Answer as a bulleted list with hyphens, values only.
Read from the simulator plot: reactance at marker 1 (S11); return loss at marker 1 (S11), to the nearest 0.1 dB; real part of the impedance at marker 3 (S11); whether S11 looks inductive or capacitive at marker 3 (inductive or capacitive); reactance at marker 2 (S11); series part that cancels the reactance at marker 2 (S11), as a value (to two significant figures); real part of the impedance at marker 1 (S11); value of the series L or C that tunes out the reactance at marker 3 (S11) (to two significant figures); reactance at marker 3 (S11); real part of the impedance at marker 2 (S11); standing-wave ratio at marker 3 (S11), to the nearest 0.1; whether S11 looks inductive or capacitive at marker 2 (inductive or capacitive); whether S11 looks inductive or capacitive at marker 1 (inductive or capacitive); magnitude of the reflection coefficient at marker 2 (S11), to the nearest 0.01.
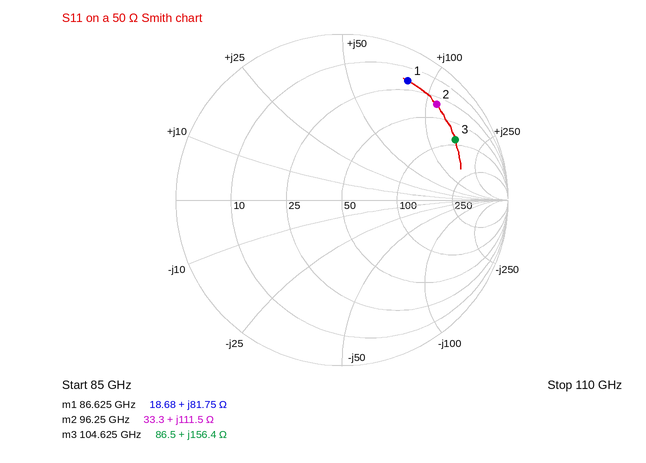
- +81.75 Ω
- 1.7 dB
- 86.5 Ω
- inductive
- +111.5 Ω
- 15 fF
- 18.68 Ω
- 9.7 fF
- +156.4 Ω
- 33.3 Ω
- 7.8
- inductive
- inductive
- 0.81
